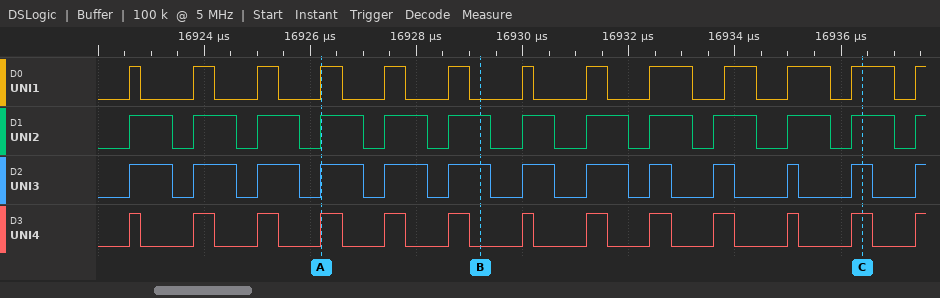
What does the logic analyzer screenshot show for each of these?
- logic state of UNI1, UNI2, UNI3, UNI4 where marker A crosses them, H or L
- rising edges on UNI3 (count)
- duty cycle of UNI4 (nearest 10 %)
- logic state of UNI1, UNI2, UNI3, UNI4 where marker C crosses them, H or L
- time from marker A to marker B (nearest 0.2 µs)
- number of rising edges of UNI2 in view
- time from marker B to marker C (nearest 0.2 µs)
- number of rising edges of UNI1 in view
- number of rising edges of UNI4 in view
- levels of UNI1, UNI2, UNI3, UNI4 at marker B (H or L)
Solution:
UNI1=H, UNI2=H, UNI3=H, UNI4=H
13
30 %
UNI1=H, UNI2=H, UNI3=H, UNI4=H
3 µs
13
7.2 µs
13
13
UNI1=L, UNI2=H, UNI3=H, UNI4=L
